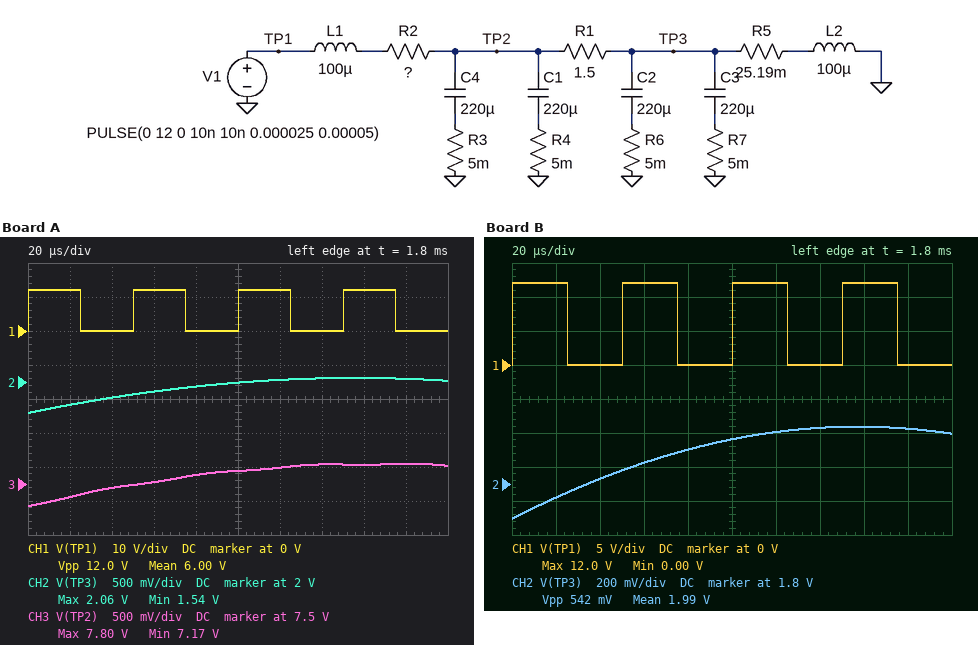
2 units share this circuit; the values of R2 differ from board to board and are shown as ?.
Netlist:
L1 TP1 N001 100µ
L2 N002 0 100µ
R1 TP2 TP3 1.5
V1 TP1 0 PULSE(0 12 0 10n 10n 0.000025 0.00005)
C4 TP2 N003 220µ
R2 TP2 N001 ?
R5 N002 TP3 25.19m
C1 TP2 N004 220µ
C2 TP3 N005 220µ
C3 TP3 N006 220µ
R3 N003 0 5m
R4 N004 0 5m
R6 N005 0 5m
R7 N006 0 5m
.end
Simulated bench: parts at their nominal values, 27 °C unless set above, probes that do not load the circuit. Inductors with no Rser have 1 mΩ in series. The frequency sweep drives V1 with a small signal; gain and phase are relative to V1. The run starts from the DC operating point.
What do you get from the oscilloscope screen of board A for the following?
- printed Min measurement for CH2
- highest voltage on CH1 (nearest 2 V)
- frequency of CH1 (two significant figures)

1.54 V
12 V
20 kHz
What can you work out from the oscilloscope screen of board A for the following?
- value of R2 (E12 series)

0.047 Ω
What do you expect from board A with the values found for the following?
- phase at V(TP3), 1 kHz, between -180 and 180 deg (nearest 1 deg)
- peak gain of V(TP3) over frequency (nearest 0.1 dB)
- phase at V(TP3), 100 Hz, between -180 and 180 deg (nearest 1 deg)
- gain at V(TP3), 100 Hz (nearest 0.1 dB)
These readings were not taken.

151 deg
14.6 dB
62 deg
-27.0 dB
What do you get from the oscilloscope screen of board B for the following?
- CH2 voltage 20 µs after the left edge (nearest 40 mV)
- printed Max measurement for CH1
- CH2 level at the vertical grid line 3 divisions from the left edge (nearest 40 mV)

1.72 V
12.0 V
1.92 V
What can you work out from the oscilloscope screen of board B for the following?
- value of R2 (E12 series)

0.039 Ω
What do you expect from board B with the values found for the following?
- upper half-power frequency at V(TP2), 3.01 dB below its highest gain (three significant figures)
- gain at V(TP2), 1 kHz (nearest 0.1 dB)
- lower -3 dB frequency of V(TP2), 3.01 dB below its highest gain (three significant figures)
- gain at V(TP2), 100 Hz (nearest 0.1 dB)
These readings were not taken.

786 Hz
0.1 dB
728 Hz
-0.1 dB
